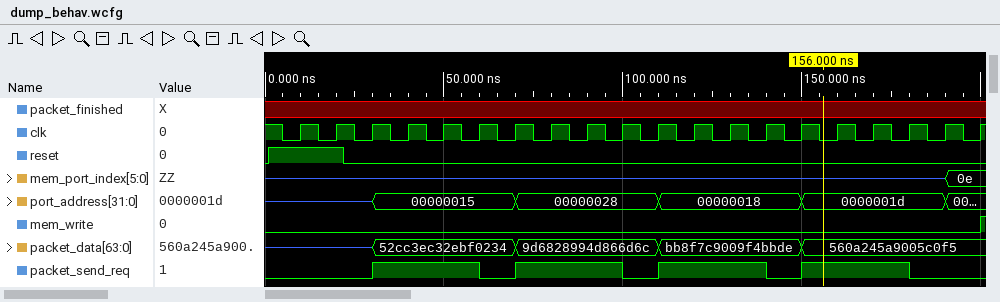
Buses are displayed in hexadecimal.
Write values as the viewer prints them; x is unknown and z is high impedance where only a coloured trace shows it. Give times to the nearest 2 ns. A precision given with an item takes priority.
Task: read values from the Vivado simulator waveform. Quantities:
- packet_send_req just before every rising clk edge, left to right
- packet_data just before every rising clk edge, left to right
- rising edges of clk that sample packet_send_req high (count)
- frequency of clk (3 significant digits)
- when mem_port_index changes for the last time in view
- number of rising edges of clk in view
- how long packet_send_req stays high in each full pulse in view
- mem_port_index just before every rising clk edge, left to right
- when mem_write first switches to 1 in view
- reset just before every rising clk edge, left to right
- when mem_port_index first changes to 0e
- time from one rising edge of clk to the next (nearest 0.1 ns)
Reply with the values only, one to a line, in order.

0 0 0 1 1 1 0 1 1 1 0 1 1 1 0 1 1 1 0 0
z, z, z, 52cc3ec32ebf0234, 52cc3ec32ebf0234, 52cc3ec32ebf0234, 52cc3ec32ebf0234, 9d6828994d866d6c, 9d6828994d866d6c, 9d6828994d866d6c, 9d6828994d866d6c, bb8f7c9009f4bbde, bb8f7c9009f4bbde, bb8f7c9009f4bbde, bb8f7c9009f4bbde, 560a245a9005c0f5, 560a245a9005c0f5, 560a245a9005c0f5, 560a245a9005c0f5, 560a245a9005c0f5
12
100 MHz
190 ns
20
30 ns, 30 ns, 30 ns, 30 ns
z, z, z, z, z, z, z, z, z, z, z, z, z, z, z, z, z, z, z, 0e
200 ns
1 1 0 0 0 0 0 0 0 0 0 0 0 0 0 0 0 0 0 0
190 ns
10 ns
